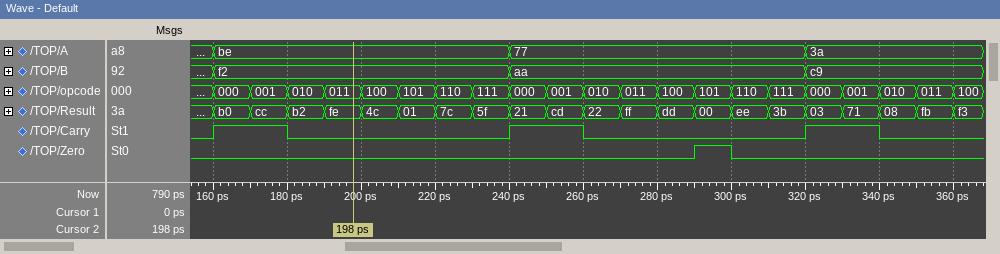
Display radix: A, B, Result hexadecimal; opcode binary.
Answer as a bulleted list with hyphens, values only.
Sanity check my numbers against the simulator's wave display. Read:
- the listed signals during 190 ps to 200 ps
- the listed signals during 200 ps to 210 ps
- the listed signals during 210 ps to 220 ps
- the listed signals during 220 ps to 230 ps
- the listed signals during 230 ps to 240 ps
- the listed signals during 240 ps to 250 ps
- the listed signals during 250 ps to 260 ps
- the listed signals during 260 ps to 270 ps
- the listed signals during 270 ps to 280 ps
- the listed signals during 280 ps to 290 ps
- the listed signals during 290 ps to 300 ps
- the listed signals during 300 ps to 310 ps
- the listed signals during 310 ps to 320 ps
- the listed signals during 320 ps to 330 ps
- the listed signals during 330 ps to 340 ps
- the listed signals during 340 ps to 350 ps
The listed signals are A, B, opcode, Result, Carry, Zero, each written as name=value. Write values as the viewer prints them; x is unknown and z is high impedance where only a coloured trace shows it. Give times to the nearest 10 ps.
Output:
- A=be, B=f2, opcode=011, Result=fe, Carry=0, Zero=0
- A=be, B=f2, opcode=100, Result=4c, Carry=0, Zero=0
- A=be, B=f2, opcode=101, Result=01, Carry=0, Zero=0
- A=be, B=f2, opcode=110, Result=7c, Carry=0, Zero=0
- A=be, B=f2, opcode=111, Result=5f, Carry=0, Zero=0
- A=77, B=aa, opcode=000, Result=21, Carry=1, Zero=0
- A=77, B=aa, opcode=001, Result=cd, Carry=1, Zero=0
- A=77, B=aa, opcode=010, Result=22, Carry=0, Zero=0
- A=77, B=aa, opcode=011, Result=ff, Carry=0, Zero=0
- A=77, B=aa, opcode=100, Result=dd, Carry=0, Zero=0
- A=77, B=aa, opcode=101, Result=00, Carry=0, Zero=1
- A=77, B=aa, opcode=110, Result=ee, Carry=0, Zero=0
- A=77, B=aa, opcode=111, Result=3b, Carry=0, Zero=0
- A=3a, B=c9, opcode=000, Result=03, Carry=1, Zero=0
- A=3a, B=c9, opcode=001, Result=71, Carry=1, Zero=0
- A=3a, B=c9, opcode=010, Result=08, Carry=0, Zero=0
